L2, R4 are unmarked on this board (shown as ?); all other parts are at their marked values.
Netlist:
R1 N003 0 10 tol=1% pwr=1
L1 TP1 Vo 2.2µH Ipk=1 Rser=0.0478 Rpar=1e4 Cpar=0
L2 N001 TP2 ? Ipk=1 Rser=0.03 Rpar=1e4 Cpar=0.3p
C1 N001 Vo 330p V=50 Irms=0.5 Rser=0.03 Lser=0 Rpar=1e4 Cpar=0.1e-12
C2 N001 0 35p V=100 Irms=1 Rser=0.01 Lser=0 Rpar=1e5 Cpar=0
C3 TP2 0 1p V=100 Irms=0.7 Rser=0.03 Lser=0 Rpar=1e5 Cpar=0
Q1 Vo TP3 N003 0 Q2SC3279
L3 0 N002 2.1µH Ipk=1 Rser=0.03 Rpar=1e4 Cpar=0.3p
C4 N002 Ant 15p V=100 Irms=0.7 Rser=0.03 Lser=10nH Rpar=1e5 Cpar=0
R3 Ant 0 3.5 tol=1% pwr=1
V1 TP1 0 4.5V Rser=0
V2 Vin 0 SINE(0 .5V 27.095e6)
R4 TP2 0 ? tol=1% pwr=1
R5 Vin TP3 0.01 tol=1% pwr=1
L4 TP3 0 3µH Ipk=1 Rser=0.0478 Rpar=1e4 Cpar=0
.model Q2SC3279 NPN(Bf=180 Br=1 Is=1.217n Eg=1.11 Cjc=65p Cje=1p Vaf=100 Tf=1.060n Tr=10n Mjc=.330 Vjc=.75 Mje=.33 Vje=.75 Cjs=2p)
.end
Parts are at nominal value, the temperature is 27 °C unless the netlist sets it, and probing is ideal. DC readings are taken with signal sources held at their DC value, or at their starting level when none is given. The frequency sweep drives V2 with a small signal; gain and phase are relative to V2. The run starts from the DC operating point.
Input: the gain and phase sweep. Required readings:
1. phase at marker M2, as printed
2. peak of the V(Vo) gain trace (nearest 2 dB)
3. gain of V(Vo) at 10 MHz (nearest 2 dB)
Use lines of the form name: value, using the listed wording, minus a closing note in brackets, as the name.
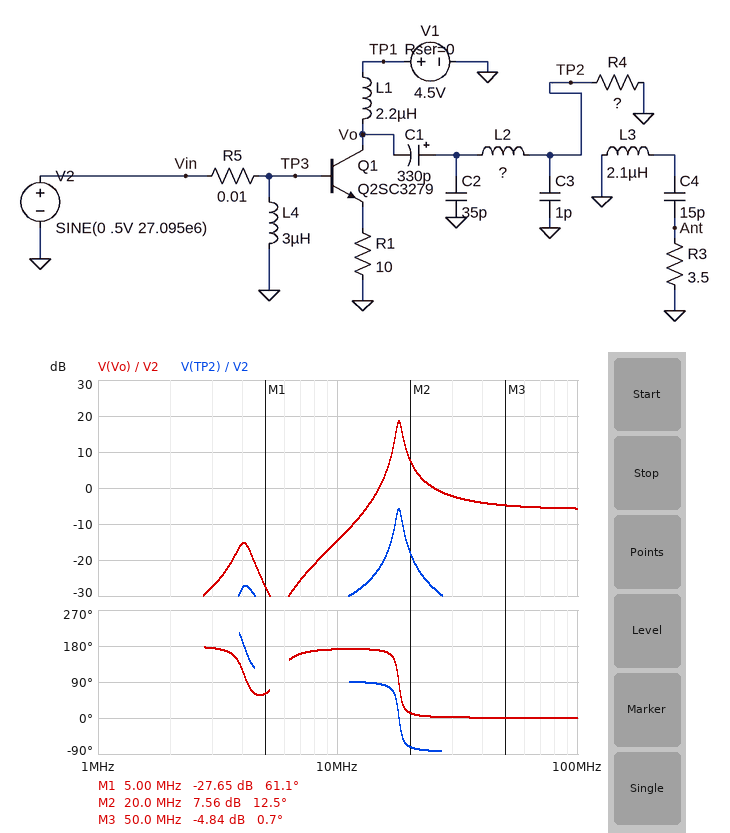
phase at marker M2, as printed: 12.5 deg
peak of the V(Vo) gain trace: 18 dB
gain of V(Vo) at 10 MHz: -14 dB
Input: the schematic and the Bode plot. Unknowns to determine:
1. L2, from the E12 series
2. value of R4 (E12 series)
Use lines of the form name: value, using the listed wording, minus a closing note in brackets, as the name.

L2, from the E12 series: 2.2 µH
value of R4: 15 Ω
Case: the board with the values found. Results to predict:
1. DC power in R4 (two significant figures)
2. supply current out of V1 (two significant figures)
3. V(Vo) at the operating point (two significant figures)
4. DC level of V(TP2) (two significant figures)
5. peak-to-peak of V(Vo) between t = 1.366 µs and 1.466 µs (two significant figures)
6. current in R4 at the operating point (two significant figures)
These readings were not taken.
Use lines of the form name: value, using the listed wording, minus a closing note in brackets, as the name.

DC power in R4: 3.0 µW
supply current out of V1: 450 µA
V(Vo) at the operating point: 4.5 V
DC level of V(TP2): 6.7 mV
peak-to-peak of V(Vo) between t = 1.366 µs and 1.466 µs: 1.3 V
current in R4 at the operating point: 450 µA
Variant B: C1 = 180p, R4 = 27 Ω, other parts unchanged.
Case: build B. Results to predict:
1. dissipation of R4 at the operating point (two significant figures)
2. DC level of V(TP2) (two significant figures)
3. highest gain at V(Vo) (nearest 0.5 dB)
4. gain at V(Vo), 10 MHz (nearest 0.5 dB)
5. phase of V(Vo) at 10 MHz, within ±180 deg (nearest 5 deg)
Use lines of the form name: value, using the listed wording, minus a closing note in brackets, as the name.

dissipation of R4 at the operating point: 5.4 µW
DC level of V(TP2): 12 mV
highest gain at V(Vo): 15.5 dB
gain at V(Vo), 10 MHz: -15.5 dB
phase of V(Vo) at 10 MHz, within ±180 deg: 160 deg
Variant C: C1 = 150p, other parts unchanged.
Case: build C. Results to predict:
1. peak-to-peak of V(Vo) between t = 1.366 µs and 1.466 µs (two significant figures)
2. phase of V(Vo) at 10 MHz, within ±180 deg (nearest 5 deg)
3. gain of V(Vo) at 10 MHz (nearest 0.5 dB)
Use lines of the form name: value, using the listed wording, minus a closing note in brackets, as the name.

peak-to-peak of V(Vo) between t = 1.366 µs and 1.466 µs: 1.4 V
phase of V(Vo) at 10 MHz, within ±180 deg: 165 deg
gain of V(Vo) at 10 MHz: -17.0 dB
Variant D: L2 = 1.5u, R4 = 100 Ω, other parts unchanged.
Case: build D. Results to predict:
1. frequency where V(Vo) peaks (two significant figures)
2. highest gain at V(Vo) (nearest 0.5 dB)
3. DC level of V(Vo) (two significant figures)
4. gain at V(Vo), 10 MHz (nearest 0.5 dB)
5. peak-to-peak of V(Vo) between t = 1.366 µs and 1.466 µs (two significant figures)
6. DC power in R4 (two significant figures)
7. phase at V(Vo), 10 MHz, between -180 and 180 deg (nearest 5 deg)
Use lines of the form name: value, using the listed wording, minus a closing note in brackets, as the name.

frequency where V(Vo) peaks: 20 MHz
highest gain at V(Vo): 4.0 dB
DC level of V(Vo): 4.5 V
gain at V(Vo), 10 MHz: -12.5 dB
peak-to-peak of V(Vo) between t = 1.366 µs and 1.466 µs: 1.4 V
DC power in R4: 20 µW
phase at V(Vo), 10 MHz, between -180 and 180 deg: 135 deg
